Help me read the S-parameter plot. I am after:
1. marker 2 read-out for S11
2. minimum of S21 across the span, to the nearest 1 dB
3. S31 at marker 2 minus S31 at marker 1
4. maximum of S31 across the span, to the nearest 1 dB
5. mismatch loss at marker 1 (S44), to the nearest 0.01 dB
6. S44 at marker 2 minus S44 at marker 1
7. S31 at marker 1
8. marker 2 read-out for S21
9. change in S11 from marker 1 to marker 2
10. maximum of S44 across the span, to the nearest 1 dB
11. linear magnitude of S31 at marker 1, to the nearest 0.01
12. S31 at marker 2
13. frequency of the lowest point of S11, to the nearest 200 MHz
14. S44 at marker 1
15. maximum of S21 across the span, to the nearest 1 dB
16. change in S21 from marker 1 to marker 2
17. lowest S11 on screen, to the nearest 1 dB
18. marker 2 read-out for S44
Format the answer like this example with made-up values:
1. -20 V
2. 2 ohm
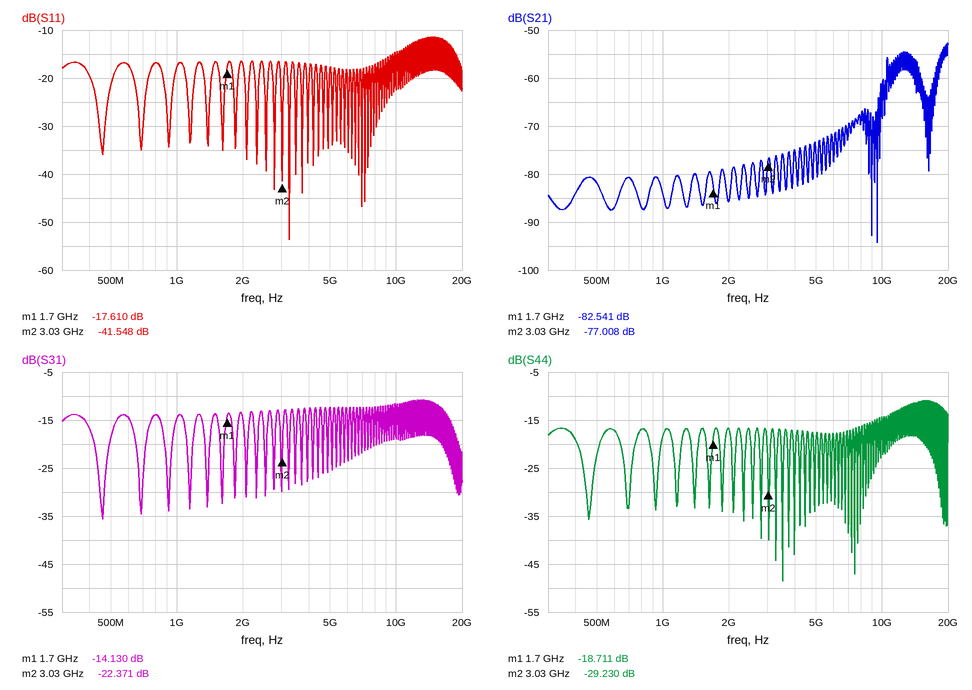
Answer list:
1. -41.548 dB
2. -94 dB
3. -8.241 dB
4. -11 dB
5. 0.06 dB
6. -10.519 dB
7. -14.130 dB
8. -77.008 dB
9. -23.938 dB
10. -11 dB
11. 0.20
12. -22.371 dB
13. 3.2 GHz
14. -18.711 dB
15. -53 dB
16. 5.533 dB
17. -54 dB
18. -29.230 dB
